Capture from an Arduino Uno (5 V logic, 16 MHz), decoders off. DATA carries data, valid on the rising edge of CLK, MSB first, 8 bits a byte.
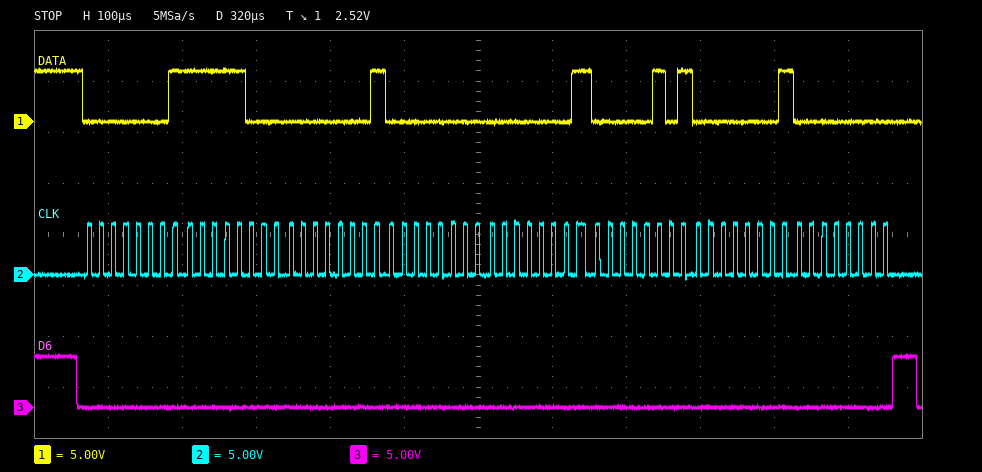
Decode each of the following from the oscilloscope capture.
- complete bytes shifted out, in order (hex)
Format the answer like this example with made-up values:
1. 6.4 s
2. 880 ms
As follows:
1. 01 F8 01 00 01 05 01 00
